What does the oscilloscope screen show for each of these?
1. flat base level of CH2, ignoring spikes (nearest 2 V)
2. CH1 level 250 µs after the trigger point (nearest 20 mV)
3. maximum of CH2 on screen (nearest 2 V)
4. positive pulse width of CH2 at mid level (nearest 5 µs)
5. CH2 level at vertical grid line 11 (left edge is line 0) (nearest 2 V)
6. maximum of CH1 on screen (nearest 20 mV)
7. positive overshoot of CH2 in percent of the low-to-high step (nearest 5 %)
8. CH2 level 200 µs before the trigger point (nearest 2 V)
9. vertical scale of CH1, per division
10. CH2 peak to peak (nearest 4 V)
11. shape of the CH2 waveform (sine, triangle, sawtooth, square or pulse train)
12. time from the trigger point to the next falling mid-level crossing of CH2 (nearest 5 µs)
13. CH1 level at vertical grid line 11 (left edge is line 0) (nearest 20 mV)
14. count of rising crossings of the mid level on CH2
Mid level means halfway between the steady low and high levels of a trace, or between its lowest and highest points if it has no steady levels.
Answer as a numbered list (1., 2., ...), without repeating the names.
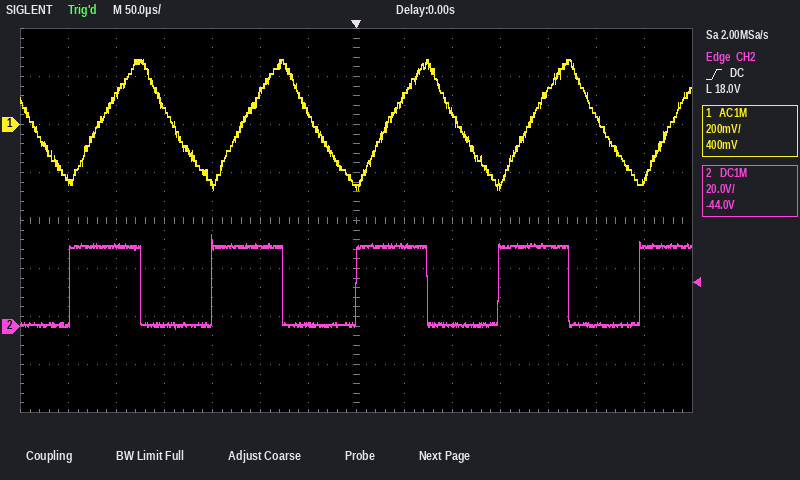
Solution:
1. 0 V
2. 40 mV
3. 38 V
4. 75 µs
5. 34 V
6. 280 mV
7. 15 %
8. 0 V
9. 200 mV
10. 40 V
11. square
12. 75 µs
13. 140 mV
14. 5
